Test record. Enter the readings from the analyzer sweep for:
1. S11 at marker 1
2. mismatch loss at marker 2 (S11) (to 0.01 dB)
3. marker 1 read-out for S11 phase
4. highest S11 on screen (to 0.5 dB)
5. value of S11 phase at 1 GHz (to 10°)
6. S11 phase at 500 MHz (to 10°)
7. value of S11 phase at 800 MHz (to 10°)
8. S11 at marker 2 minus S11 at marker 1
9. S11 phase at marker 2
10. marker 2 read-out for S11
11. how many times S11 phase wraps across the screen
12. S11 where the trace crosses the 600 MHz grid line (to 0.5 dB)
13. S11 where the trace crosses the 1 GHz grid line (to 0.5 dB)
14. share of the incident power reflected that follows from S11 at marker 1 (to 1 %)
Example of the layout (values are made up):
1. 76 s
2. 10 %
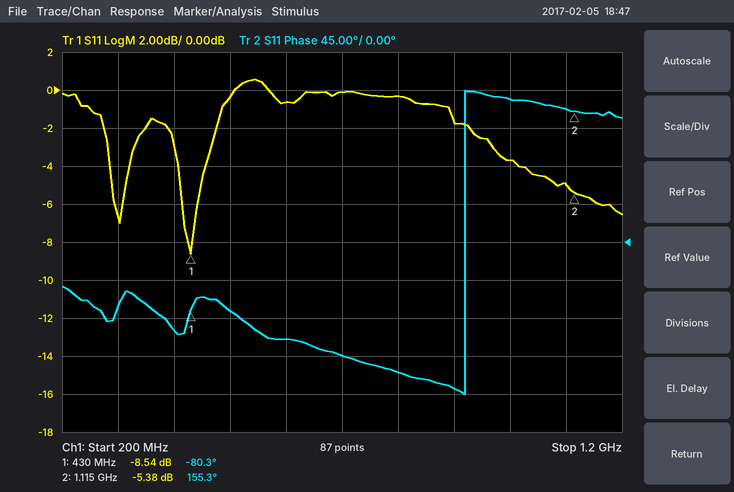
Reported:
1. -8.54 dB
2. 1.49 dB
3. -80.3°
4. 0.5 dB
5. 170°
6. -80°
7. -150°
8. 3.16 dB
9. 155.3°
10. -5.38 dB
11. 1
12. -0.5 dB
13. -3.5 dB
14. 14 %
